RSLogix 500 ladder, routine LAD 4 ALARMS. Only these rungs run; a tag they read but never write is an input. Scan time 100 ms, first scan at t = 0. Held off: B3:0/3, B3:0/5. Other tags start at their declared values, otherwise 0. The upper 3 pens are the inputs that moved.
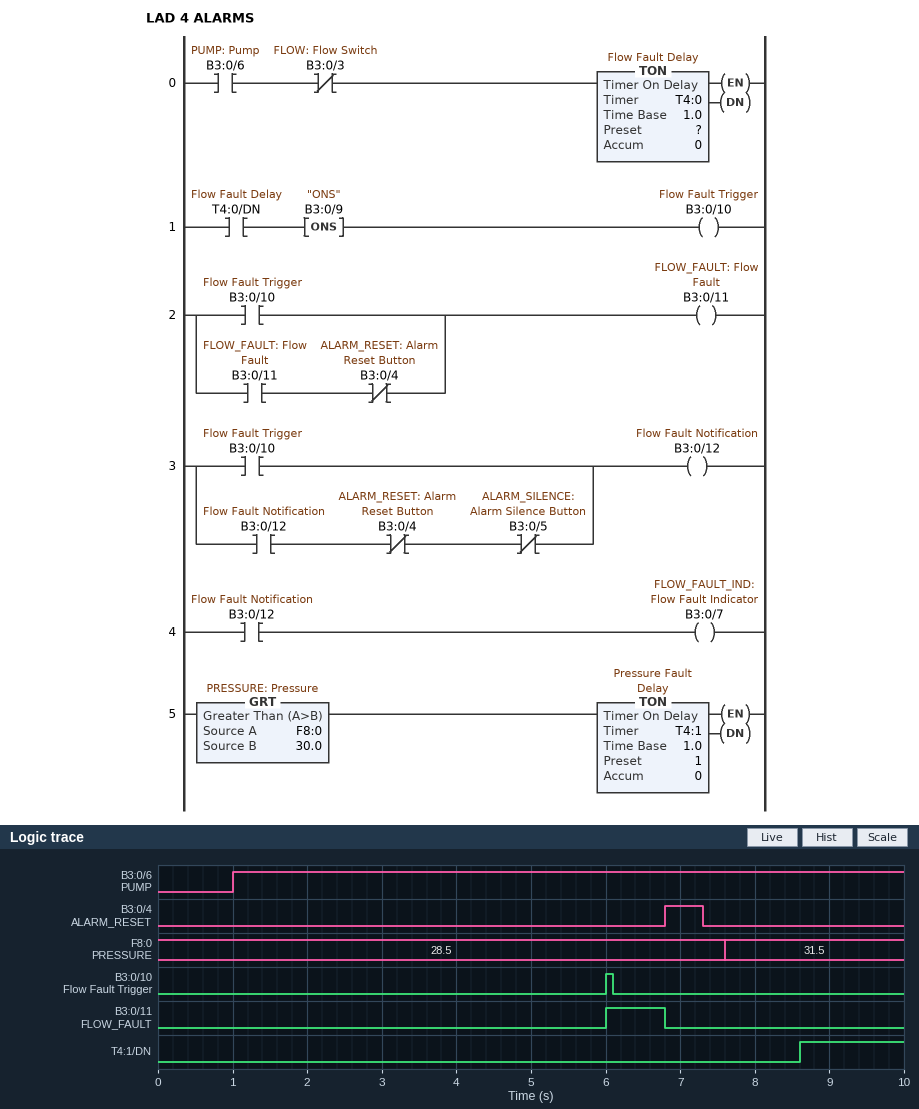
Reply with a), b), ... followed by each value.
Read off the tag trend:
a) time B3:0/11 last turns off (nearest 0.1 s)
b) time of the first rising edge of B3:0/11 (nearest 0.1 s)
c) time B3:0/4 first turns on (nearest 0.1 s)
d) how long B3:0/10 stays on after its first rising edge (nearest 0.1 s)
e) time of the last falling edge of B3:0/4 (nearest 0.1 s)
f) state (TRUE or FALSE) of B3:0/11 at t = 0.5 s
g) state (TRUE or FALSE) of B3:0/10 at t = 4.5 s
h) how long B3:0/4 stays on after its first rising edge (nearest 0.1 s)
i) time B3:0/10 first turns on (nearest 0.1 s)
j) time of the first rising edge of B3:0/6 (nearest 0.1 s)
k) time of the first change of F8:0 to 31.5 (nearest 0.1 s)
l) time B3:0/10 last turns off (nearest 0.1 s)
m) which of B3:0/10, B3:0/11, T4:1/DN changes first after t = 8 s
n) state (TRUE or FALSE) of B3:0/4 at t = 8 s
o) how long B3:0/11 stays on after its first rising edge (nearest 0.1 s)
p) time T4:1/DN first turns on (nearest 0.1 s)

a) 6.8 s
b) 6.0 s
c) 6.8 s
d) 0.1 s
e) 7.3 s
f) FALSE
g) FALSE
h) 0.5 s
i) 6.0 s
j) 1.0 s
k) 7.6 s
l) 6.1 s
m) T4:1/DN
n) FALSE
o) 0.8 s
p) 8.6 s
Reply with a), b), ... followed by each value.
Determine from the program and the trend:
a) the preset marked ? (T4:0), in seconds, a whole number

a) 5 s
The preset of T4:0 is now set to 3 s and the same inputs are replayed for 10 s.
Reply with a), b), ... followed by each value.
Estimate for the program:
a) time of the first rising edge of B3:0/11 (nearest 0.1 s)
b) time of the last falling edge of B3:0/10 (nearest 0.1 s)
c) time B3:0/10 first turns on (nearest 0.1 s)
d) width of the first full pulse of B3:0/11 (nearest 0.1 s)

a) 4.0 s
b) 4.1 s
c) 4.0 s
d) 2.8 s
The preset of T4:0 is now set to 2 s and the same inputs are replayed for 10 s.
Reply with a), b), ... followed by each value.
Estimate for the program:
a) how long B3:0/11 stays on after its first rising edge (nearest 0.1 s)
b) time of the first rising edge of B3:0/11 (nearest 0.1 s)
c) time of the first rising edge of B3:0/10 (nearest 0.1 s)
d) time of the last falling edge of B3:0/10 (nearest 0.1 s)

a) 3.8 s
b) 3.0 s
c) 3.0 s
d) 3.1 s
